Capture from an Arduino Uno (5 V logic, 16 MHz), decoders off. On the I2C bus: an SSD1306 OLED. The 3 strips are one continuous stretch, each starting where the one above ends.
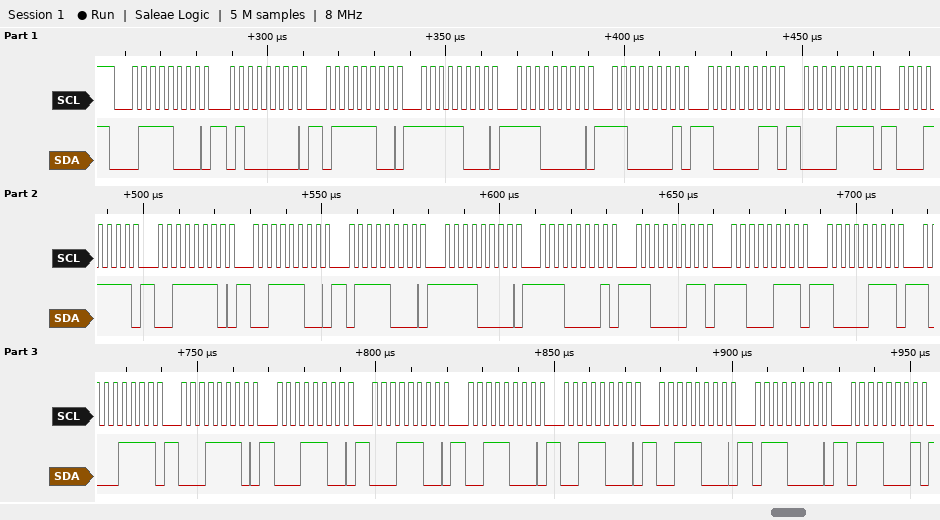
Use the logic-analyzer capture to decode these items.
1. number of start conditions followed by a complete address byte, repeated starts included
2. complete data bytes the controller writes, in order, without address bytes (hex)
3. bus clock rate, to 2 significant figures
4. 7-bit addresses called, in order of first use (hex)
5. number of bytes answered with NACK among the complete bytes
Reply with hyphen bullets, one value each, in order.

- 1
- 40 7C F8 E0 C1 83 0F 1F 3E 3C 78 F0 E1 C3 C7 87 8F 1E 1C 1C 38 38 38 70 71
- 400 kHz
- 0x3C
- 0
